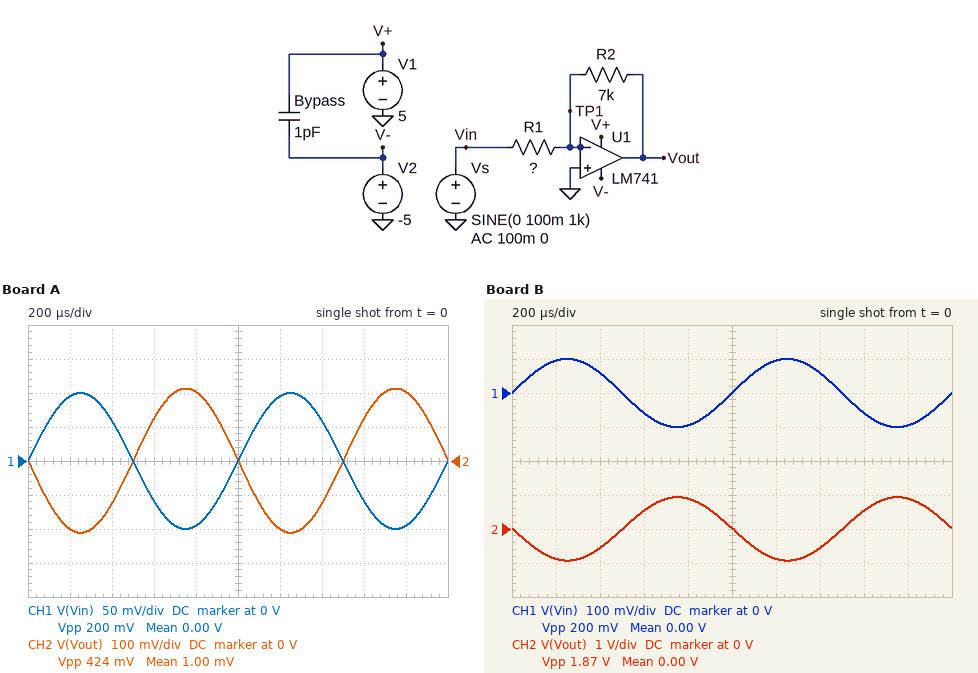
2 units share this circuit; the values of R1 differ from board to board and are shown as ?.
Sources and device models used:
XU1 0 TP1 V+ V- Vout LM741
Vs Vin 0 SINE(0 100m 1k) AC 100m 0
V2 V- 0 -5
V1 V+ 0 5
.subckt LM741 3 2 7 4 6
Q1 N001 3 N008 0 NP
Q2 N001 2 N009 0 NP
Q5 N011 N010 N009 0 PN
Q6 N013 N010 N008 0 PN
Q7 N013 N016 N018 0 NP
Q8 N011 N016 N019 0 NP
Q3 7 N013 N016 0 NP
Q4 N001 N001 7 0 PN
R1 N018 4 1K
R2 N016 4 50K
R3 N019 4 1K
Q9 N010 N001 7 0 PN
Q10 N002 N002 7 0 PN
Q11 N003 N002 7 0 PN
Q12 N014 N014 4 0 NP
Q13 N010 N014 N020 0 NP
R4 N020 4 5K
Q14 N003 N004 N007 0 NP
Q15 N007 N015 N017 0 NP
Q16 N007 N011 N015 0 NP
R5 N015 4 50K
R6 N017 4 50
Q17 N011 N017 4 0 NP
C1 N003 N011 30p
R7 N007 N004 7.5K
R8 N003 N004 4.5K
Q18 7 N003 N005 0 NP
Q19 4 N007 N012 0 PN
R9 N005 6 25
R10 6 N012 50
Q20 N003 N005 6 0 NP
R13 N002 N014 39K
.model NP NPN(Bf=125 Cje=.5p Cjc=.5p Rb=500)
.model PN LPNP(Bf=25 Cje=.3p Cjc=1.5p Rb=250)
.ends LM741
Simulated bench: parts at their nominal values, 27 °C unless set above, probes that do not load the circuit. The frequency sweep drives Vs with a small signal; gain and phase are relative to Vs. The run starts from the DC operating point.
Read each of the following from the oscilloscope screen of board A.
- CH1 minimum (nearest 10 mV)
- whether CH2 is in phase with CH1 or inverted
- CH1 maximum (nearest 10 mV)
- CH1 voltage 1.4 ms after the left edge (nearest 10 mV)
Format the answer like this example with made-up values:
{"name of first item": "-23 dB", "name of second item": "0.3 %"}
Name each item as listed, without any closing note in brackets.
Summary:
{"CH1 minimum": "-100 mV", "whether CH2 is in phase with CH1 or inverted": "inverted", "CH1 maximum": "100 mV", "CH1 voltage 1.4 ms after the left edge": "60 mV"}
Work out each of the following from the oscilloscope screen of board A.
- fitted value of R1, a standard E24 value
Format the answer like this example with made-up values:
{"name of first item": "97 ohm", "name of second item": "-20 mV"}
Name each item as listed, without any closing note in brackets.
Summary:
{"fitted value of R1, a standard E24 value": "3.3 kΩ"}
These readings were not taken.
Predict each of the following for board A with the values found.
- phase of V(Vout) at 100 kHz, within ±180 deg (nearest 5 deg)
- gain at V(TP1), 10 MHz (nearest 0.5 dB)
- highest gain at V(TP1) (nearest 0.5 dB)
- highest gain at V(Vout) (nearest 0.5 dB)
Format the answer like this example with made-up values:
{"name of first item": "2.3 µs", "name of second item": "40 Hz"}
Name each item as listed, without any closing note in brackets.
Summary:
{"phase of V(Vout) at 100 kHz, within ±180 deg": "95 deg", "gain at V(TP1), 10 MHz": "-1.5 dB", "highest gain at V(TP1)": "-1.0 dB", "highest gain at V(Vout)": "6.5 dB"}
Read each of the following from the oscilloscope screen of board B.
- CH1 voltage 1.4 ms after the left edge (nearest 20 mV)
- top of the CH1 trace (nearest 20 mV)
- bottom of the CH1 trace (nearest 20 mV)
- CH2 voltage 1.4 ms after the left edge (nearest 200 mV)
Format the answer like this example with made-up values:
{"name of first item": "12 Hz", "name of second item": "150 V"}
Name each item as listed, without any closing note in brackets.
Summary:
{"CH1 voltage 1.4 ms after the left edge": "60 mV", "top of the CH1 trace": "100 mV", "bottom of the CH1 trace": "-100 mV", "CH2 voltage 1.4 ms after the left edge": "-600 mV"}
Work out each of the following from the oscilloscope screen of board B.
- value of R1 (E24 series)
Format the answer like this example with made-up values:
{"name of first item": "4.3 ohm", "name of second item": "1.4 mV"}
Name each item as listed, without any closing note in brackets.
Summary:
{"value of R1": "750 Ω"}
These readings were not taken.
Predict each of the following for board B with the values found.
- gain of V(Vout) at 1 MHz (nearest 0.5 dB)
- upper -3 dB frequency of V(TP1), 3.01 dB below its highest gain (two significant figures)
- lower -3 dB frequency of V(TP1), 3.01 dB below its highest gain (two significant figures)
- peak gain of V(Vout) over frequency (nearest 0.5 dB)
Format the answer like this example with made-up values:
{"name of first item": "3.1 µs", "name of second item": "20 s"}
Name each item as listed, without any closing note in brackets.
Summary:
{"gain of V(Vout) at 1 MHz": "-2.5 dB", "upper -3 dB frequency of V(TP1), 3.01 dB below its highest gain": "280 MHz", "lower -3 dB frequency of V(TP1), 3.01 dB below its highest gain": "16 kHz", "peak gain of V(Vout) over frequency": "19.5 dB"}
